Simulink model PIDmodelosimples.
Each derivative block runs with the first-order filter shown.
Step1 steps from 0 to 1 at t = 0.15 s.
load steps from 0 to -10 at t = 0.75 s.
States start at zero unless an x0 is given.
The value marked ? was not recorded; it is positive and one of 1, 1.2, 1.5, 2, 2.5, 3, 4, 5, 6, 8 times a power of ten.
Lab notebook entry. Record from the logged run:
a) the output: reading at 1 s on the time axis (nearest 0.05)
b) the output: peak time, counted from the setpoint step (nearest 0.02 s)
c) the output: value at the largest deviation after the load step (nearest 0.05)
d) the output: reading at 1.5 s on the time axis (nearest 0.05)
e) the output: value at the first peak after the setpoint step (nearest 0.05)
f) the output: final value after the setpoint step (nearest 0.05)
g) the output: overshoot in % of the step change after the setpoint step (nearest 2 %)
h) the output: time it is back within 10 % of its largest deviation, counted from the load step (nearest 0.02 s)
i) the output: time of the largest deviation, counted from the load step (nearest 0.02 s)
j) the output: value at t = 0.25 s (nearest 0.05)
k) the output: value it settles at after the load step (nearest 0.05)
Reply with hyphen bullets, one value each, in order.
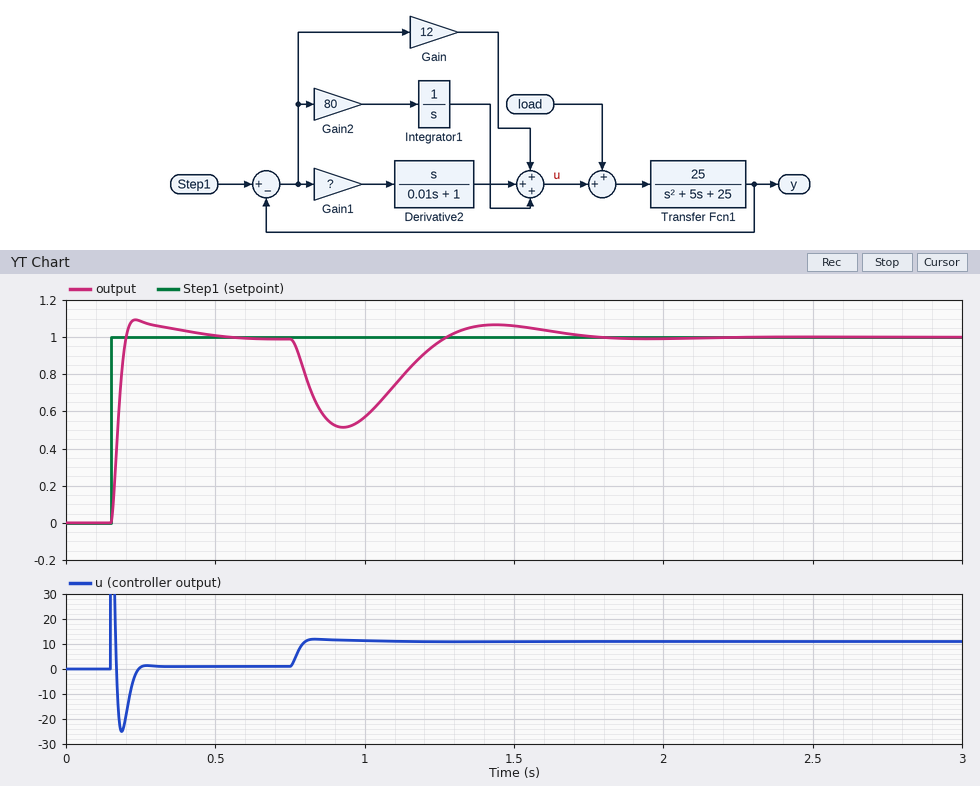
- 0.55
- 0.08 s
- 0.50
- 1.05
- 1.10
- 1.00
- 10 %
- 0.82 s
- 0.18 s
- 1.10
- 1.00
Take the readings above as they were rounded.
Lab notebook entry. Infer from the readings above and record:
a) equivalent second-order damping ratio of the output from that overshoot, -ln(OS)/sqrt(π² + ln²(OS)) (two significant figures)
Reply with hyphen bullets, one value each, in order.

- 0.59
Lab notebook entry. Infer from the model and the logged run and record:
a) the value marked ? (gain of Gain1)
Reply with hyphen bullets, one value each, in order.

- 1.5
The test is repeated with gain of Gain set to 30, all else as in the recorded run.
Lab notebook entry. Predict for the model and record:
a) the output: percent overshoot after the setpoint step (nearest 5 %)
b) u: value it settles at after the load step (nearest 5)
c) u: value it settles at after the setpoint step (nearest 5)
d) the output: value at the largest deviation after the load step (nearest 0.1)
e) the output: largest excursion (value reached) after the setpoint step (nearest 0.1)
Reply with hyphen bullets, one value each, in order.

- 25 %
- 10
- 0
- 0.7
- 1.2
